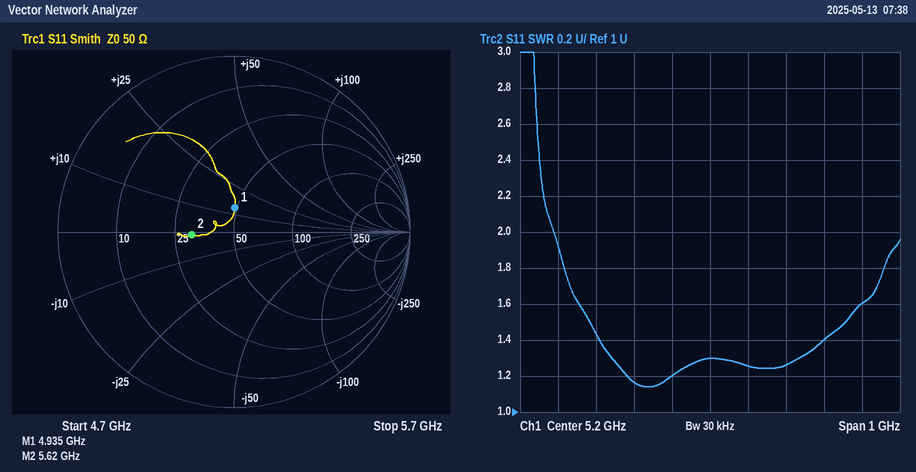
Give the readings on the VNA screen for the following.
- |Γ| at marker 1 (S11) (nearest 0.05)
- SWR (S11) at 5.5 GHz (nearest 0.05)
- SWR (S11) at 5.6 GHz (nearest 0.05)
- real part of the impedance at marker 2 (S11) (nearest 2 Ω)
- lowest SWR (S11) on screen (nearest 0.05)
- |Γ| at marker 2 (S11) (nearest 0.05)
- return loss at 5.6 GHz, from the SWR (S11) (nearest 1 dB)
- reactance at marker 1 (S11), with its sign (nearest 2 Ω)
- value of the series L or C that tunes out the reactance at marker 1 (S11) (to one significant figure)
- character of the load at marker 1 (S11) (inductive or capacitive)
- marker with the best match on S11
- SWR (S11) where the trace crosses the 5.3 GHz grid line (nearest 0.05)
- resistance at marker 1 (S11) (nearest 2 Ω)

0.15
1.40
1.60
30 Ω
1.15
0.25
13 dB
+14 Ω
2 pF
inductive
marker 1
1.25
48 Ω
